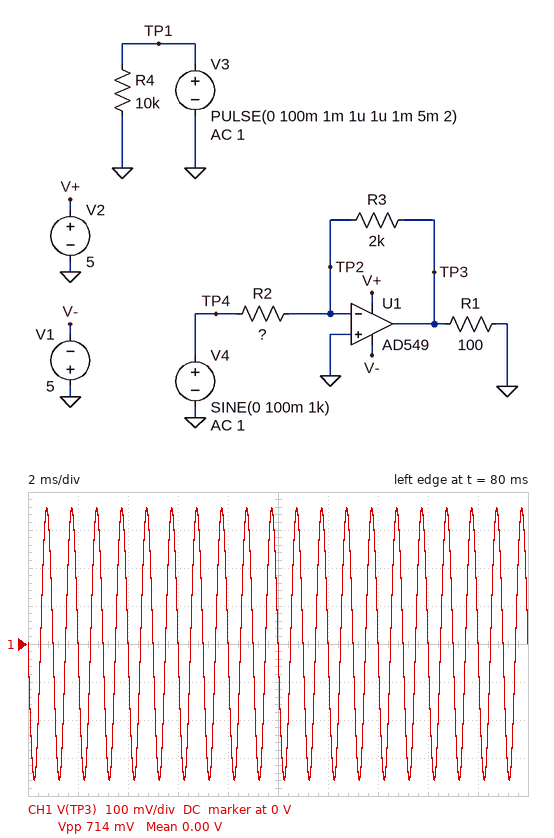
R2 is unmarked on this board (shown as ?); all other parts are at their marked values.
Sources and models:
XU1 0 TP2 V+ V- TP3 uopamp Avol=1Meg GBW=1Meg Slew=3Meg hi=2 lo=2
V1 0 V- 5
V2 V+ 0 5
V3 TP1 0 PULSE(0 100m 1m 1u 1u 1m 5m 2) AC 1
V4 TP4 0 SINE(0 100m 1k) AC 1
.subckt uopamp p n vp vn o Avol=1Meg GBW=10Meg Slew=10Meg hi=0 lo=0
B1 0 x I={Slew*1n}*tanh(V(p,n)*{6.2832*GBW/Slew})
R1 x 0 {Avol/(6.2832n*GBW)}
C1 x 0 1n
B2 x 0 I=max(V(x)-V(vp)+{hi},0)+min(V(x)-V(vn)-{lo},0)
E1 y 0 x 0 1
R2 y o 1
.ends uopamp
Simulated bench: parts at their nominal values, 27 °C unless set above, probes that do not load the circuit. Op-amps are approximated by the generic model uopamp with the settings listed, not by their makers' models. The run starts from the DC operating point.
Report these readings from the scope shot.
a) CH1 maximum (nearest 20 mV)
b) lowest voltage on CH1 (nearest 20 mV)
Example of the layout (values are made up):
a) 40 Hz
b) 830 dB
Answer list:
a) 360 mV
b) -360 mV
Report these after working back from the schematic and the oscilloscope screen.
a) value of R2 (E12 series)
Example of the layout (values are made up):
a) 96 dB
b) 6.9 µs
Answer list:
a) 560 Ω
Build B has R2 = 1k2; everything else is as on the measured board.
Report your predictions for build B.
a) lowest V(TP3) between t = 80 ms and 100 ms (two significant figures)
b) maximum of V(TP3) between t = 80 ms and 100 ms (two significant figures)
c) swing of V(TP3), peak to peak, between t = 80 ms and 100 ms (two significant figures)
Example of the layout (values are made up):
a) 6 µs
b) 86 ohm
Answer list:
a) -170 mV
b) 170 mV
c) 330 mV
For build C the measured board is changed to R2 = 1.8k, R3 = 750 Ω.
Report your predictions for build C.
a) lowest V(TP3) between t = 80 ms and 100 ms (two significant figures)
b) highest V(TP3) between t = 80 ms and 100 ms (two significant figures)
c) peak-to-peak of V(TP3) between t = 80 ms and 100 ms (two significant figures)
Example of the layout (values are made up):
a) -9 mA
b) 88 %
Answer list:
a) -42 mV
b) 42 mV
c) 83 mV
